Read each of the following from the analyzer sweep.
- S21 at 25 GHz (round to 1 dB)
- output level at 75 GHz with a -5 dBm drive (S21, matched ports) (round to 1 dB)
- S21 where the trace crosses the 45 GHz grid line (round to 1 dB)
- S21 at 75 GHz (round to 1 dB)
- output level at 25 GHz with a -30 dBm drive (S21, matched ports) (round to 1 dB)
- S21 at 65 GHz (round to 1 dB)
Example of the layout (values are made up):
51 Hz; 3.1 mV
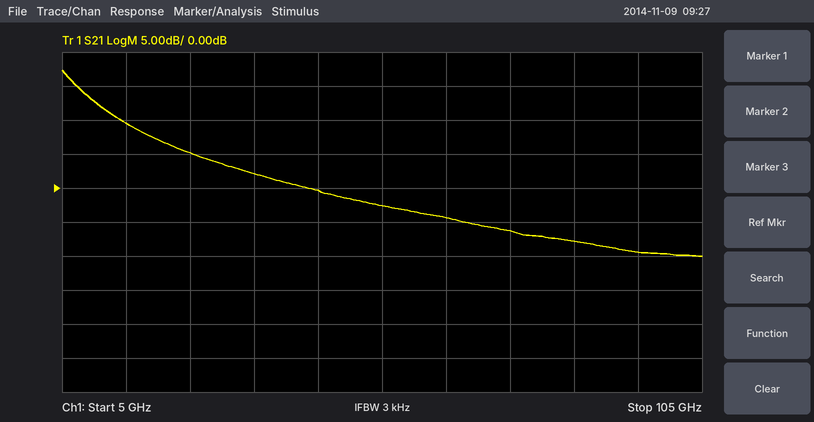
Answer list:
5 dB; -11 dBm; 0 dB; -6 dB; -25 dBm; -4 dB
